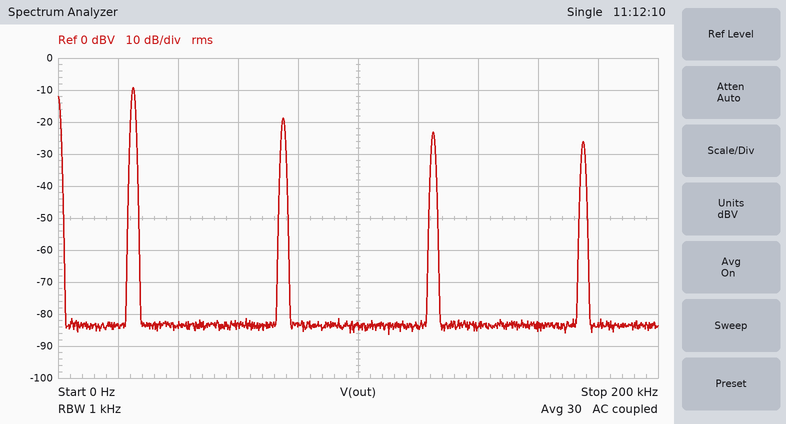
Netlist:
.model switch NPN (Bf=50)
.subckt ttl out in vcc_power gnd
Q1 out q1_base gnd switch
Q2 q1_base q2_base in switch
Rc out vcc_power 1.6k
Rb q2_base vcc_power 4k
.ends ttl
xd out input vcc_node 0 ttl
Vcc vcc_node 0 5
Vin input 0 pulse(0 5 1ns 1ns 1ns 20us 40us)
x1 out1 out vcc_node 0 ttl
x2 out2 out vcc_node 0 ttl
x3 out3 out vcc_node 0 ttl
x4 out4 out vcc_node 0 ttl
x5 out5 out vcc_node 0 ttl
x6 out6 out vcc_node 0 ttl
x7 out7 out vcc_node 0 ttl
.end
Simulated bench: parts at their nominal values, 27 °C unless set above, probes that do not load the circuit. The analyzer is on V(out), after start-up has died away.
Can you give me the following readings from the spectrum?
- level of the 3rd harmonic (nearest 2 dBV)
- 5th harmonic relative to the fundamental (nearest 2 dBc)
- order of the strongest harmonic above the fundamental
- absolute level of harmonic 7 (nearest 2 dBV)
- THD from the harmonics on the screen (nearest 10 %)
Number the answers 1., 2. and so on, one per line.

1. -18 dBV
2. -14 dBc
3. 3
4. -26 dBV
5. 40 %
